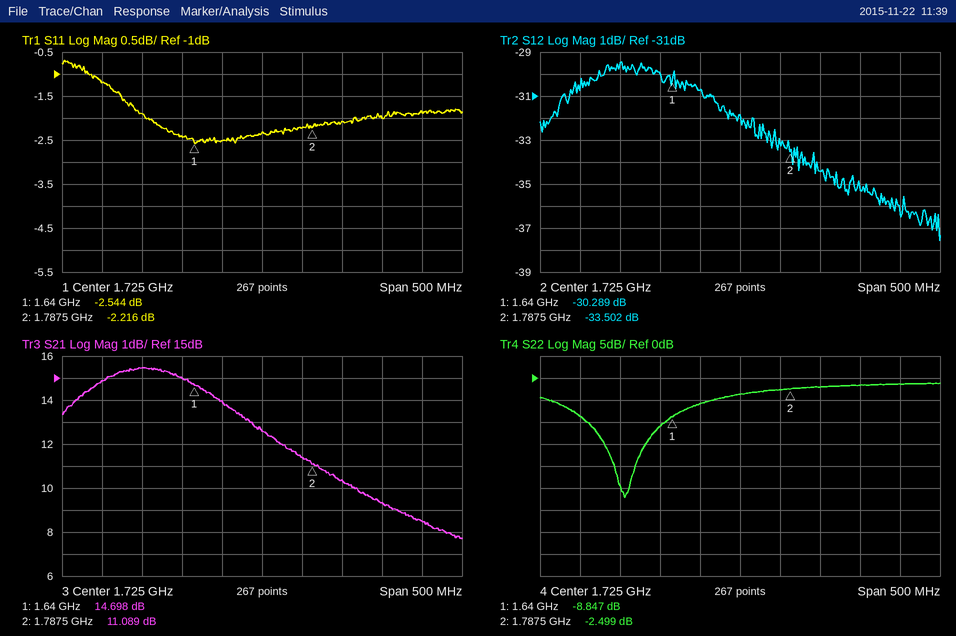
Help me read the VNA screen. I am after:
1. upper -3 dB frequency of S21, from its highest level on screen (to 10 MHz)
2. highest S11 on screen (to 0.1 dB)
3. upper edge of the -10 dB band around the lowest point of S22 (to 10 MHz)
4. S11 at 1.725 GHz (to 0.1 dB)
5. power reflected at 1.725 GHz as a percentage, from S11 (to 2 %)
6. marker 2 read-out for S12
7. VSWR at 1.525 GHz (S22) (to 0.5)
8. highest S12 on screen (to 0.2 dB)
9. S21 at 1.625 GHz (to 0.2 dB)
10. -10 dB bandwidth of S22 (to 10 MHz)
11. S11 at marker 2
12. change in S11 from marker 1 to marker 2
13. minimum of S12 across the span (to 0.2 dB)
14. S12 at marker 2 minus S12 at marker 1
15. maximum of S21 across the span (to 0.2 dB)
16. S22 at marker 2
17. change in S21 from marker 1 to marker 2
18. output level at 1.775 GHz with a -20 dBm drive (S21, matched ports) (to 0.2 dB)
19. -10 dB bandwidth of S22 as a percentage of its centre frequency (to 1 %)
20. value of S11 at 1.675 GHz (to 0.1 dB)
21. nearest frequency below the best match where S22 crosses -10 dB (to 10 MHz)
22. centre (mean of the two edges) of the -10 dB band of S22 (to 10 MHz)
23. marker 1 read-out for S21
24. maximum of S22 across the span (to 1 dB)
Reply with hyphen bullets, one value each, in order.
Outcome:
- 1.73 GHz
- -0.7 dB
- 1.63 GHz
- -2.3 dB
- 58 %
- -33.502 dB
- 2.0
- -29.4 dB
- 15.0 dB
- 100 MHz
- -2.216 dB
- 0.328 dB
- -37.6 dB
- -3.213 dB
- 15.4 dB
- -2.499 dB
- -3.609 dB
- -8.6 dBm
- 6 %
- -2.5 dB
- 1.53 GHz
- 1.58 GHz
- 14.698 dB
- -1 dB
